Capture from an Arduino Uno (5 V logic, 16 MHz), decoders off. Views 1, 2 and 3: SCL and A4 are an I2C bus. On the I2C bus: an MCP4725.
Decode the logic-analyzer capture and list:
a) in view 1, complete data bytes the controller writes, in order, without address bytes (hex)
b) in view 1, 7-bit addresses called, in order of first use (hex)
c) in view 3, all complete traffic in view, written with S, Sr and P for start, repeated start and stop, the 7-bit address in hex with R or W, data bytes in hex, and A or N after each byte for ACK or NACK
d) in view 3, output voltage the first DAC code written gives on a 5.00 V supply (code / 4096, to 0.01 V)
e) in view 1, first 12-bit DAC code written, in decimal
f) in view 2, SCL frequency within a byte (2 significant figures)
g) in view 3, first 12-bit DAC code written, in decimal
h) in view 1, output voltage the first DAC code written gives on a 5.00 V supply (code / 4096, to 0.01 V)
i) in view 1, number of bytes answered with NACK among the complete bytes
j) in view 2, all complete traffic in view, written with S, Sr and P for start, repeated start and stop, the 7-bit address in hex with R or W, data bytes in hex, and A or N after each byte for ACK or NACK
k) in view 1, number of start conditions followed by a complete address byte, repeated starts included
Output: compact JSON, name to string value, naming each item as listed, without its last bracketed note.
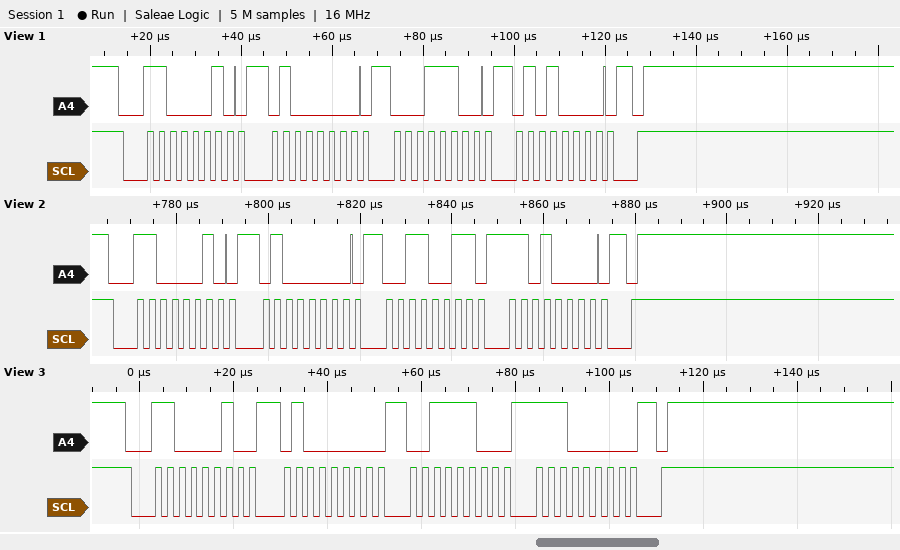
{"in view 1, complete data bytes the controller writes, in order, without address bytes": "40 1C 50", "in view 1, 7-bit addresses called, in order of first use": "0x61", "in view 3, all complete traffic in view, written with S, Sr and P for start, repeated start and stop, the 7-bit address in hex with R or W, data bytes in hex, and A or N after each byte for ACK or NACK": "S 61W A 40 A 3C A E0 A P", "in view 3, output voltage the first DAC code written gives on a 5.00 V supply": "1.19 V", "in view 1, first 12-bit DAC code written, in decimal": "453", "in view 2, SCL frequency within a byte": "400 kHz", "in view 3, first 12-bit DAC code written, in decimal": "974", "in view 1, output voltage the first DAC code written gives on a 5.00 V supply": "0.55 V", "in view 1, number of bytes answered with NACK among the complete bytes": "0", "in view 2, all complete traffic in view, written with S, Sr and P for start, repeated start and stop, the 7-bit address in hex with R or W, data bytes in hex, and A or N after each byte for ACK or NACK": "S 61W A 40 A 33 A D0 A P", "in view 1, number of start conditions followed by a complete address byte, repeated starts included": "1"}
